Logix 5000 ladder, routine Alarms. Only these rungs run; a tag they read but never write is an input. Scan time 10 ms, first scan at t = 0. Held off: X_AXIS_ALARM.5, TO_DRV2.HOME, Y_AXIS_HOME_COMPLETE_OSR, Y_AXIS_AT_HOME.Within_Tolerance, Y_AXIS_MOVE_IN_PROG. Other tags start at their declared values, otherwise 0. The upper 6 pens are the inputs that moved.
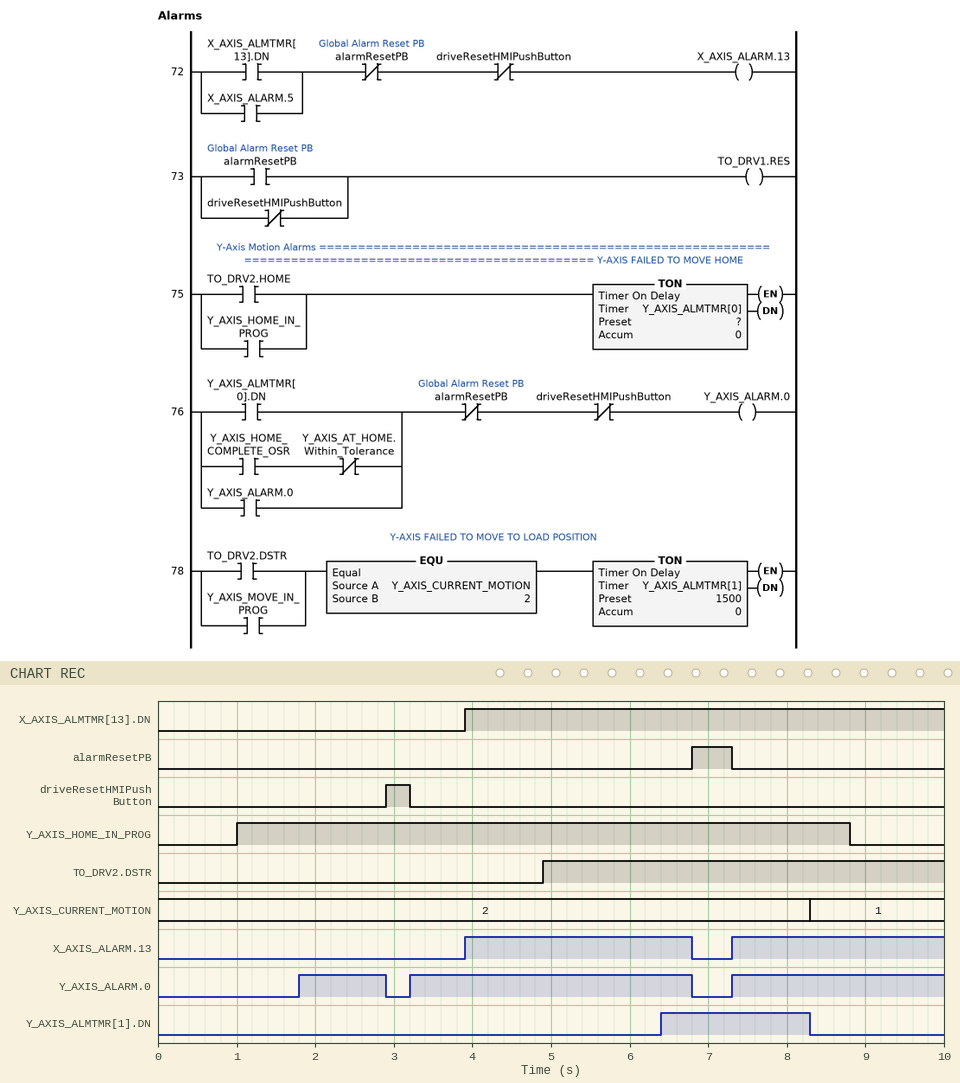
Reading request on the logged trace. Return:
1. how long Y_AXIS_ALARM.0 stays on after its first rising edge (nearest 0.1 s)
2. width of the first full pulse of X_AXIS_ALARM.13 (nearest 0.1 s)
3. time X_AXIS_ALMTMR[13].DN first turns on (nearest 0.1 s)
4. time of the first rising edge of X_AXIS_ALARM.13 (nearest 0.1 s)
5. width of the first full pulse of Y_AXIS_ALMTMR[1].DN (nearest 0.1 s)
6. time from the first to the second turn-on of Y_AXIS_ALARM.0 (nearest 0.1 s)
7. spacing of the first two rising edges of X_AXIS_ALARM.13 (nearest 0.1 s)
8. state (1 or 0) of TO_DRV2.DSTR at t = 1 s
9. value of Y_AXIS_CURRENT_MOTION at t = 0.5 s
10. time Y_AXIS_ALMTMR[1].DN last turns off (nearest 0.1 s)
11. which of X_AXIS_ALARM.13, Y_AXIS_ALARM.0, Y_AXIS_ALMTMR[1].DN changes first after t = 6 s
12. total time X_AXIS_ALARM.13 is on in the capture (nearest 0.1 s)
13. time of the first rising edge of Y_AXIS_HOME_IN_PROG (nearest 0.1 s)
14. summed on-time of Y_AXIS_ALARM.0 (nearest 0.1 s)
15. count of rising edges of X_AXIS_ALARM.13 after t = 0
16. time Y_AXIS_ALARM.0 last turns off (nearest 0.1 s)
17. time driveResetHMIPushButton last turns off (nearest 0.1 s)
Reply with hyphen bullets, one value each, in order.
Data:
- 1.1 s
- 2.9 s
- 3.9 s
- 3.9 s
- 1.9 s
- 1.4 s
- 3.4 s
- 0
- 2
- 8.3 s
- Y_AXIS_ALMTMR[1].DN
- 5.6 s
- 1.0 s
- 7.4 s
- 2
- 6.8 s
- 3.2 s
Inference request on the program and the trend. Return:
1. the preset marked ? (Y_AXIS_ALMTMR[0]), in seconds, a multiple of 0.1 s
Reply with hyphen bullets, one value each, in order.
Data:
- 0.8 s
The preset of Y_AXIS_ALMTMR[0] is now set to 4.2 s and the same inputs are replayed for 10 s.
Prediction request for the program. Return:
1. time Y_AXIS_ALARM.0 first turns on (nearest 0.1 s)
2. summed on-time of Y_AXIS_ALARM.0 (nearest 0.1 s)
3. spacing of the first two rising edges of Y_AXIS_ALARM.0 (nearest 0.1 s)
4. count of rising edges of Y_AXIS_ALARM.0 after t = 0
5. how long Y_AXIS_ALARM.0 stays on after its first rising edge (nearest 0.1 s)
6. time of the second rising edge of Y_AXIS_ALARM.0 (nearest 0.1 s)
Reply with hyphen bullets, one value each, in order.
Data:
- 5.2 s
- 4.3 s
- 2.1 s
- 2
- 1.6 s
- 7.3 s
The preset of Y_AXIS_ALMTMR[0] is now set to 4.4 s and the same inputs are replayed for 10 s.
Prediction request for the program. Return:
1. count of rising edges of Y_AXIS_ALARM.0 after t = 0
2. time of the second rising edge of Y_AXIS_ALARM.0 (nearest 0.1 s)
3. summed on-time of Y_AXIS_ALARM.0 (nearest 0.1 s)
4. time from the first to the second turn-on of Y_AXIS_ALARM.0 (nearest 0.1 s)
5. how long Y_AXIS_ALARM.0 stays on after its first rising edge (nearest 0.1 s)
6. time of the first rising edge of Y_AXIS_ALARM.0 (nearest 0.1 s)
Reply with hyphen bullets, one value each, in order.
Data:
- 2
- 7.3 s
- 4.1 s
- 1.9 s
- 1.4 s
- 5.4 s
